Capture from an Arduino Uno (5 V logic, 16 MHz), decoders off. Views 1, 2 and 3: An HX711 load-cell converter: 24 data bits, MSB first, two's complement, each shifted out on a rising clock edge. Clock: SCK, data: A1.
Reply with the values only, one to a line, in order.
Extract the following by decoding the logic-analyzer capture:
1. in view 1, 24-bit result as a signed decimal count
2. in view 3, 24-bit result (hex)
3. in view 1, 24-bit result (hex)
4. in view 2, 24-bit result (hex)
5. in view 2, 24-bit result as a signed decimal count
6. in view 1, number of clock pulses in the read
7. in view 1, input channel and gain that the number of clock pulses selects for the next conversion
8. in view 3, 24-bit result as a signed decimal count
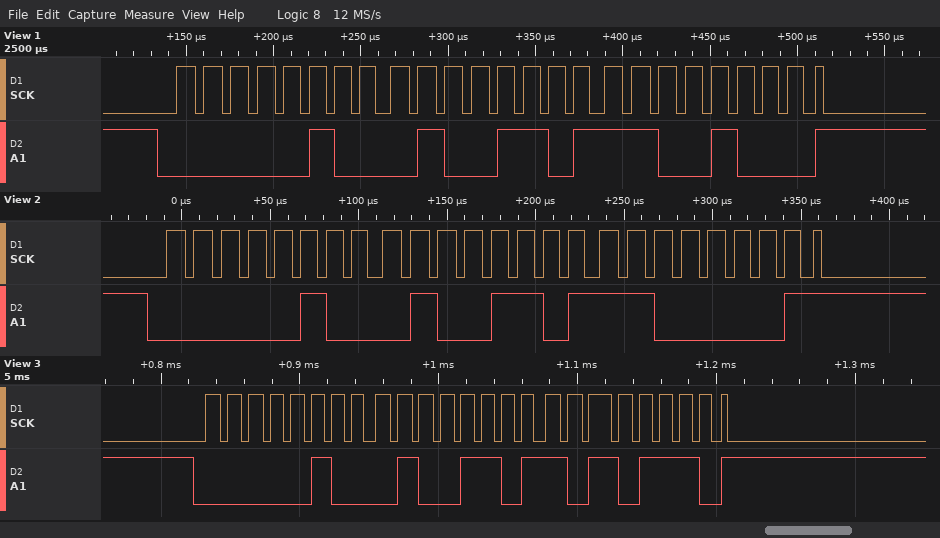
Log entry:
282056
0x044DAE
0x044DC8
0x044DC1
282049
25
channel A, gain 128
282030
